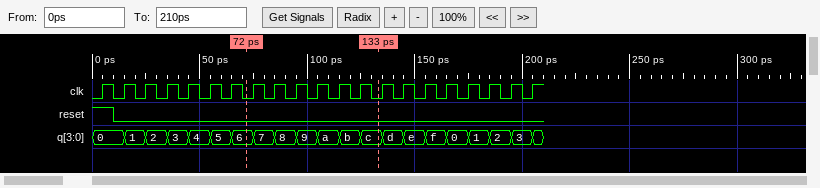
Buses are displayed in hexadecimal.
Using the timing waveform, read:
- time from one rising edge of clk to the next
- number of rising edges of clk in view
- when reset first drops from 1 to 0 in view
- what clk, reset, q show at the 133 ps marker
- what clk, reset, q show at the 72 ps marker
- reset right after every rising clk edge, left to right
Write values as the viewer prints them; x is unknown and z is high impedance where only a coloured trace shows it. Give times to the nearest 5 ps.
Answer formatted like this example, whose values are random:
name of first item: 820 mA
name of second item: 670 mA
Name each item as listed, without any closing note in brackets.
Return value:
time from one rising edge of clk to the next: 10 ps
number of rising edges of clk in view: 21
when reset first drops from 1 to 0 in view: 10 ps
what clk, reset, q show at the 133 ps marker: clk=0, reset=0, q=c
what clk, reset, q show at the 72 ps marker: clk=0, reset=0, q=6
reset right after every rising clk edge, left to right: 1 0 0 0 0 0 0 0 0 0 0 0 0 0 0 0 0 0 0 0 0
